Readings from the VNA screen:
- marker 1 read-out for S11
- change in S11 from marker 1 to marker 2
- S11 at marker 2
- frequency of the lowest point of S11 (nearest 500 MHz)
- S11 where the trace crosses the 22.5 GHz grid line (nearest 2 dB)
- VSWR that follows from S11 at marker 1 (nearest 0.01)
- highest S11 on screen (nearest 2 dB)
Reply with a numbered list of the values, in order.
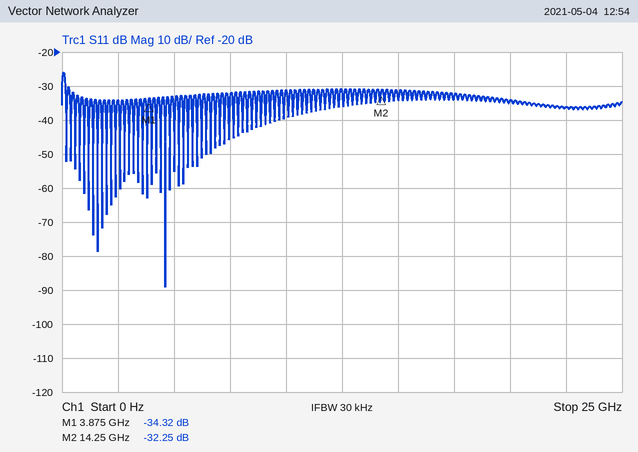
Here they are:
1. -34.32 dB
2. 2.07 dB
3. -32.25 dB
4. 4.5 GHz
5. -36 dB
6. 1.04
7. -26 dB
